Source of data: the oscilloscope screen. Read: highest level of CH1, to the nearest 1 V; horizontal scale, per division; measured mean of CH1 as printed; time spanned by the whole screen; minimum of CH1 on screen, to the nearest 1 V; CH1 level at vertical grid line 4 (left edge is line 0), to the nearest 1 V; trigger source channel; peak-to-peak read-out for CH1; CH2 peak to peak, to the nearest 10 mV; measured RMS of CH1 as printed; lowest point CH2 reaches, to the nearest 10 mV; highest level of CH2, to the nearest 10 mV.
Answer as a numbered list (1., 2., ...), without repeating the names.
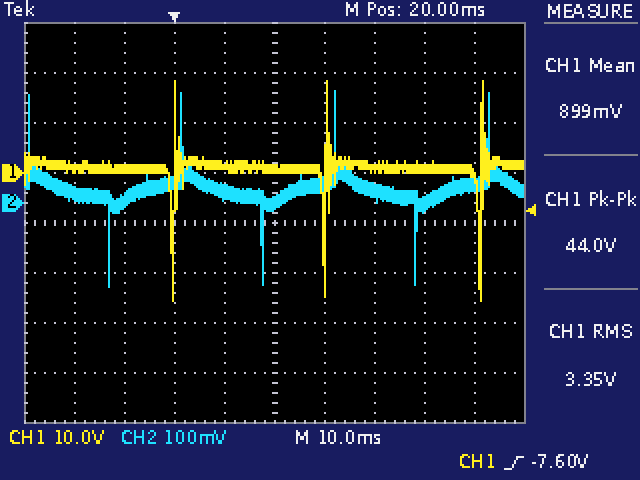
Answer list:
1. 18 V
2. 10 ms
3. 899 mV
4. 100 ms
5. -26 V
6. 2 V
7. CH1
8. 44.0 V
9. 390 mV
10. 3.35 V
11. -170 mV
12. 220 mV
